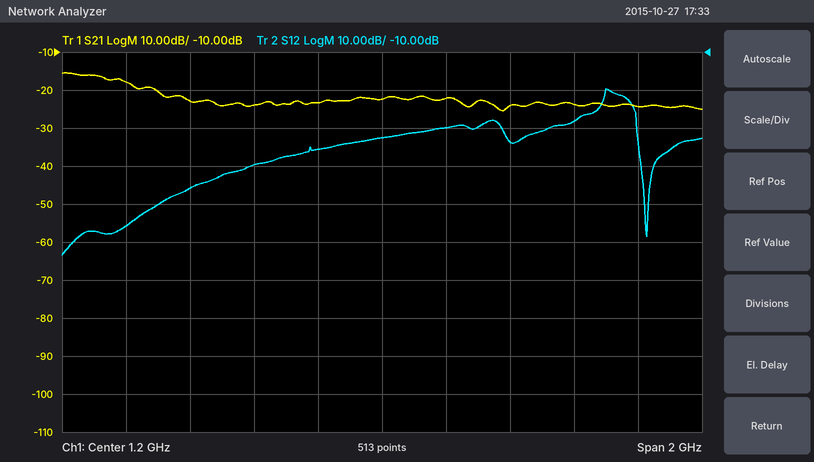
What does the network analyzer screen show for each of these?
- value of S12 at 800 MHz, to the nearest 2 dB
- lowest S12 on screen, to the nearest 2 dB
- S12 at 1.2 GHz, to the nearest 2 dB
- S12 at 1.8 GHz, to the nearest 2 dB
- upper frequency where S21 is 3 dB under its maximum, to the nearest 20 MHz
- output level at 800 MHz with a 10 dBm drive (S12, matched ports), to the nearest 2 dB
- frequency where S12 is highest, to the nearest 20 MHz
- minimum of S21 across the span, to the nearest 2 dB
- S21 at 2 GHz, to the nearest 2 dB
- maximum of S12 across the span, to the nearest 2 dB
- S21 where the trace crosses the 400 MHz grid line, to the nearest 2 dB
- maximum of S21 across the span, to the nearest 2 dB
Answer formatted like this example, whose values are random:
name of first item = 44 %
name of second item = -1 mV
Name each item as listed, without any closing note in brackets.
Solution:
value of S12 at 800 MHz, to the nearest 2 dB = -40 dB
lowest S12 on screen, to the nearest 2 dB = -64 dB
S12 at 1.2 GHz, to the nearest 2 dB = -32 dB
S12 at 1.8 GHz, to the nearest 2 dB = -28 dB
upper frequency where S21 is 3 dB under its maximum, to the nearest 20 MHz = 420 MHz
output level at 800 MHz with a 10 dBm drive (S12, matched ports), to the nearest 2 dB = -30 dBm
frequency where S12 is highest, to the nearest 20 MHz = 1.90 GHz
minimum of S21 across the span, to the nearest 2 dB = -26 dB
S21 at 2 GHz, to the nearest 2 dB = -24 dB
maximum of S12 across the span, to the nearest 2 dB = -20 dB
S21 where the trace crosses the 400 MHz grid line, to the nearest 2 dB = -18 dB
maximum of S21 across the span, to the nearest 2 dB = -16 dB
